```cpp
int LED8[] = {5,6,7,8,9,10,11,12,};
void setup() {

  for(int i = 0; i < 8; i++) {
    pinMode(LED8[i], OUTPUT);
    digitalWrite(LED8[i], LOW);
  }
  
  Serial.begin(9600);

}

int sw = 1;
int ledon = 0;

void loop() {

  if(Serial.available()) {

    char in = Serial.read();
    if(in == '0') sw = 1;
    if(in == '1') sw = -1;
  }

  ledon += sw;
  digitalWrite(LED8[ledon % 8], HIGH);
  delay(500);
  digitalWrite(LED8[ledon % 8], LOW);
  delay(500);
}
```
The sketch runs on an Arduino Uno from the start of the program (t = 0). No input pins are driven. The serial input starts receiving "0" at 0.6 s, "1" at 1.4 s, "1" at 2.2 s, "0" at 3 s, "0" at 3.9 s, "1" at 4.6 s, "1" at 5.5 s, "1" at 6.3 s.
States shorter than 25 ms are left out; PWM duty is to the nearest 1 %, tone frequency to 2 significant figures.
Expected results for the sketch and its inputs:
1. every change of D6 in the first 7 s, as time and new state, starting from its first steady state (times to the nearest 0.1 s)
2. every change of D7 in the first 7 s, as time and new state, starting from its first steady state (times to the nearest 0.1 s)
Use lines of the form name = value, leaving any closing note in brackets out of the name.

every change of D6 in the first 7 s, as time and new state, starting from its first steady state = 0 s high; 0.5 s low; 2 s high; 2.5 s low; 4 s high; 4.5 s low; 6 s high; 6.5 s low
every change of D7 in the first 7 s, as time and new state, starting from its first steady state = 0 s low; 1 s high; 1.5 s low; 5 s high; 5.5 s low
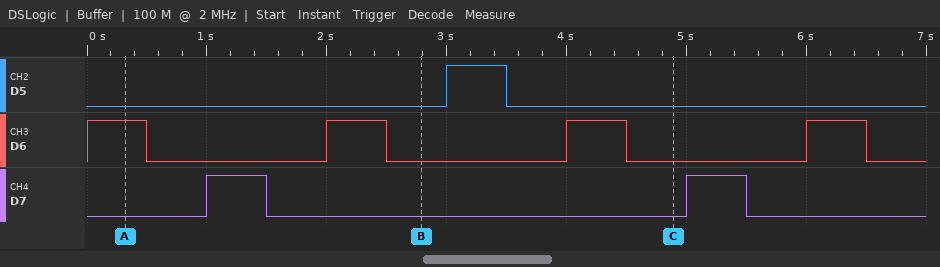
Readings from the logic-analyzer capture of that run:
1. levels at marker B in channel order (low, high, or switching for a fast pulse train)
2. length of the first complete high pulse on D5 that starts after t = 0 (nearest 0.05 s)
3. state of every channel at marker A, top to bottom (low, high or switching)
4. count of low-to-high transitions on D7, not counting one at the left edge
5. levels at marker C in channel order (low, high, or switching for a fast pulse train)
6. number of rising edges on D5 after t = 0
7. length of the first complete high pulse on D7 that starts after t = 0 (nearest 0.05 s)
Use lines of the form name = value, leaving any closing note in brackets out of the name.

levels at marker B in channel order = D5 low, D6 low, D7 low
length of the first complete high pulse on D5 that starts after t = 0 = 0.50 s
state of every channel at marker A, top to bottom = D5 low, D6 high, D7 low
count of low-to-high transitions on D7, not counting one at the left edge = 2
levels at marker C in channel order = D5 low, D6 low, D7 low
number of rising edges on D5 after t = 0 = 1
length of the first complete high pulse on D7 that starts after t = 0 = 0.50 s
